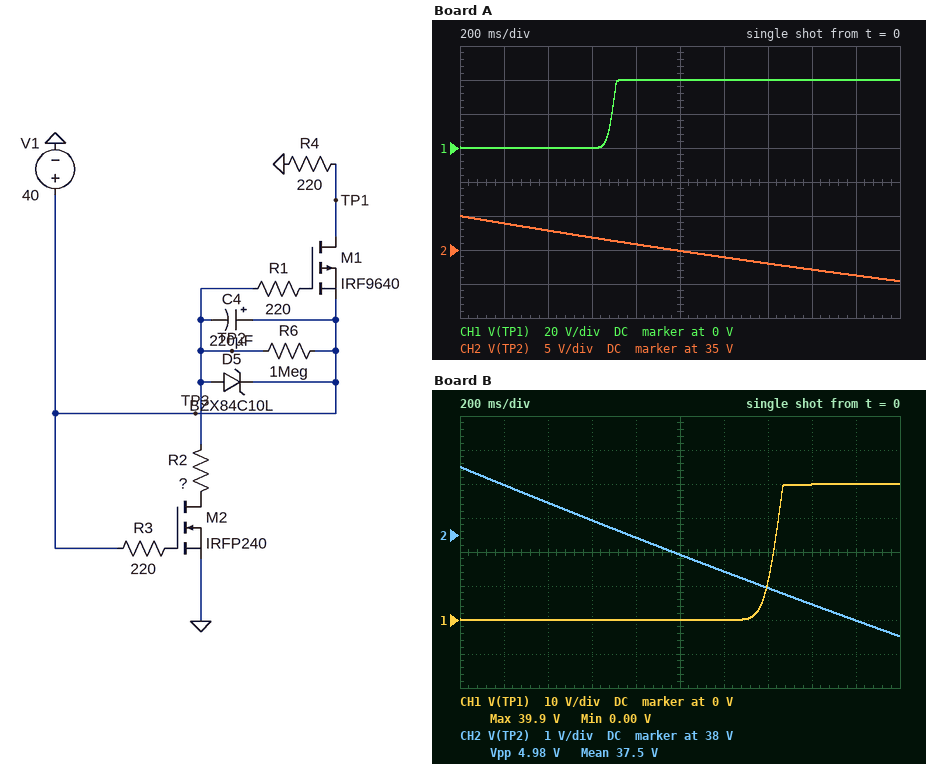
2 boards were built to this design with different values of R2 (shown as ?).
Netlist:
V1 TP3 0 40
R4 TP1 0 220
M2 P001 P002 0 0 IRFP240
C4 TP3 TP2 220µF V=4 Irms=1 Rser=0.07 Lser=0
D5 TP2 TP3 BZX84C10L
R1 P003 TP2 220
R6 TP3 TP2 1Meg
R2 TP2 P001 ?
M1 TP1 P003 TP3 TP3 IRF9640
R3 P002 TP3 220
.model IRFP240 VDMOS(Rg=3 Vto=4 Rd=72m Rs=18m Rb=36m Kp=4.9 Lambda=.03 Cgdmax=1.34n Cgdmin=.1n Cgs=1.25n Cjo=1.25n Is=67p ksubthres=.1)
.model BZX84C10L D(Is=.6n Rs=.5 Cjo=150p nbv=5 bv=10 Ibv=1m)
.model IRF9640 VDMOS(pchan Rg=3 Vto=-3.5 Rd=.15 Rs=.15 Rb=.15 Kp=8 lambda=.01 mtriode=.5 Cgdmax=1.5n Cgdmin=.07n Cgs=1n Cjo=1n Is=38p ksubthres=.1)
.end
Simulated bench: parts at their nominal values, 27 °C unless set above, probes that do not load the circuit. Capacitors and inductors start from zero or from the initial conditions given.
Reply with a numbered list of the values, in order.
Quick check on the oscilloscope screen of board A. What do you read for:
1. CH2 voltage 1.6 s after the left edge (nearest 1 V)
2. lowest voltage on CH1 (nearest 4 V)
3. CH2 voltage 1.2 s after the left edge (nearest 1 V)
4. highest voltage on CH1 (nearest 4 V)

1. 32 V
2. 0 V
3. 34 V
4. 40 V
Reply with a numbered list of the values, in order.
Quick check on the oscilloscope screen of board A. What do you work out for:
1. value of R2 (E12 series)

1. 33 kΩ
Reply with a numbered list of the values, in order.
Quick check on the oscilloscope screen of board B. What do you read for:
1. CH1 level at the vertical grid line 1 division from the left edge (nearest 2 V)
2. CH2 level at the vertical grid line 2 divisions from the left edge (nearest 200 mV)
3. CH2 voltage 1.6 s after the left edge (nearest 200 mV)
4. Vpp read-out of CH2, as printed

1. 0 V
2. 39.0 V
3. 36.0 V
4. 4.98 V
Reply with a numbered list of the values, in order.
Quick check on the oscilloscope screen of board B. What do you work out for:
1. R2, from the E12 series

1. 68 kΩ
